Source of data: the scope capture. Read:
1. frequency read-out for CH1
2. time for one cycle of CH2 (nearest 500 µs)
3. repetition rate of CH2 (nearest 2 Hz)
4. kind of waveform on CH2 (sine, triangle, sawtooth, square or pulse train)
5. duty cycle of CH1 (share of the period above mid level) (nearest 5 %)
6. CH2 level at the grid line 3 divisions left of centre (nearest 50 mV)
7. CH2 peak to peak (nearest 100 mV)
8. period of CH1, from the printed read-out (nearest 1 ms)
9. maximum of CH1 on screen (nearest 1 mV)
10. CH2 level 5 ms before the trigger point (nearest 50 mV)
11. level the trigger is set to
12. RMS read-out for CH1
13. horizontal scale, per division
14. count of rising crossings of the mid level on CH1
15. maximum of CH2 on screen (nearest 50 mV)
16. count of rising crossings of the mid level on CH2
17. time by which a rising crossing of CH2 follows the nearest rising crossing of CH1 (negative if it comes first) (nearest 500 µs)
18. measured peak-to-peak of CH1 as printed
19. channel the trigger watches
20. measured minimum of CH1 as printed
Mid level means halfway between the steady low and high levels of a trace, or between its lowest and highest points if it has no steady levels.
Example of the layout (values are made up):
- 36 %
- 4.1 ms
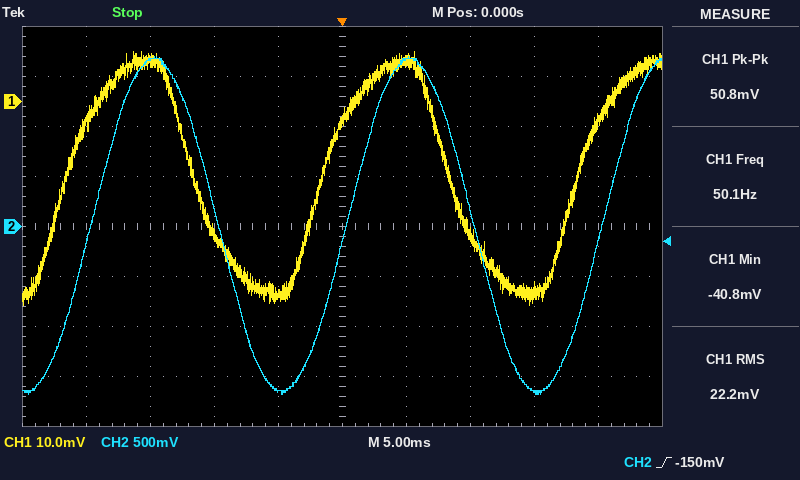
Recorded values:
- 50.1 Hz
- 20.0 ms
- 50 Hz
- sine
- 50 %
- 1.65 V
- 3.40 V
- 20 ms
- 10 mV
- -1.65 V
- -150 mV
- 22.2 mV
- 5 ms
- 3
- 1.70 V
- 3
- +2.0 ms
- 50.8 mV
- CH2
- -40.8 mV
